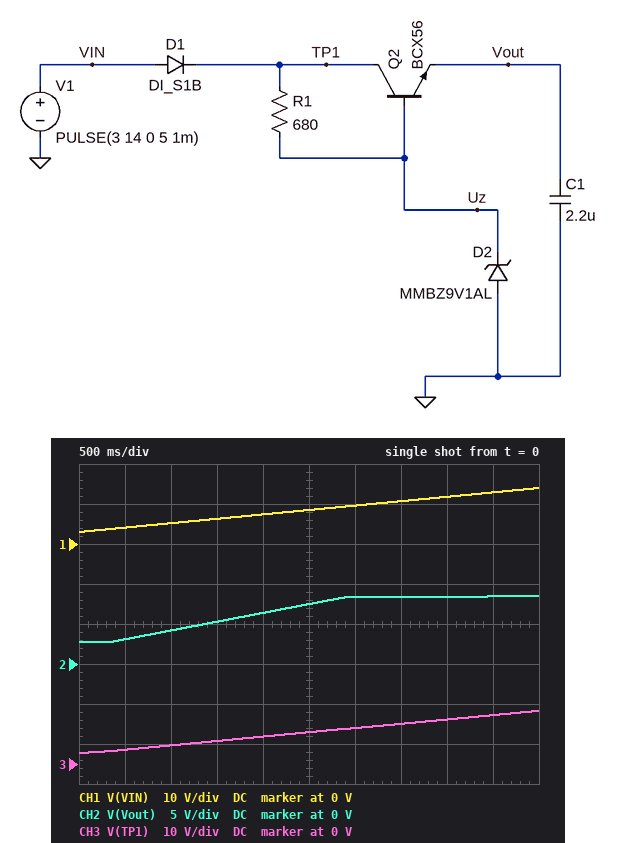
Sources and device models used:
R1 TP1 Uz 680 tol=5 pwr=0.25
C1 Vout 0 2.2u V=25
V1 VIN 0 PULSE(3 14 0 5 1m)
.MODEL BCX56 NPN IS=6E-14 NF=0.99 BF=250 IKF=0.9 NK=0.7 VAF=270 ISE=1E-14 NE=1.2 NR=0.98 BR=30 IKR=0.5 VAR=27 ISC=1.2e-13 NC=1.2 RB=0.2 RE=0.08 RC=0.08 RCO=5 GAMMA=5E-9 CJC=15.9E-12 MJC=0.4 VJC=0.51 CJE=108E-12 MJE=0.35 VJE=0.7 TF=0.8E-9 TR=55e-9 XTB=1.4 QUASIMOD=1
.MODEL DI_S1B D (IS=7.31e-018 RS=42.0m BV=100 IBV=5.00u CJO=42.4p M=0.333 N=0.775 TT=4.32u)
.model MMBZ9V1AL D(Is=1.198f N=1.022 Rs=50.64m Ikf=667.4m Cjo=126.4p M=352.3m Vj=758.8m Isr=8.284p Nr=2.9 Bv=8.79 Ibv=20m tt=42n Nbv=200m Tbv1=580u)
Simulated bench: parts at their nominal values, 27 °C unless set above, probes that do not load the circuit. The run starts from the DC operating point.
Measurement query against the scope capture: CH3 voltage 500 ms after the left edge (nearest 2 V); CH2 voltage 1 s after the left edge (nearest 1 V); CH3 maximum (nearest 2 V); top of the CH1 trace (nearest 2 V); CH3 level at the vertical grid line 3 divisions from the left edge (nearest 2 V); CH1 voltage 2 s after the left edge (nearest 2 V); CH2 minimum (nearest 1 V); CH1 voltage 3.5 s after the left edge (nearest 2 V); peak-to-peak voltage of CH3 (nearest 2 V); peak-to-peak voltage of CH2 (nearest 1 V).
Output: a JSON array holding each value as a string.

["4 V", "4 V", "14 V", "14 V", "6 V", "8 V", "3 V", "10 V", "10 V", "6 V"]
